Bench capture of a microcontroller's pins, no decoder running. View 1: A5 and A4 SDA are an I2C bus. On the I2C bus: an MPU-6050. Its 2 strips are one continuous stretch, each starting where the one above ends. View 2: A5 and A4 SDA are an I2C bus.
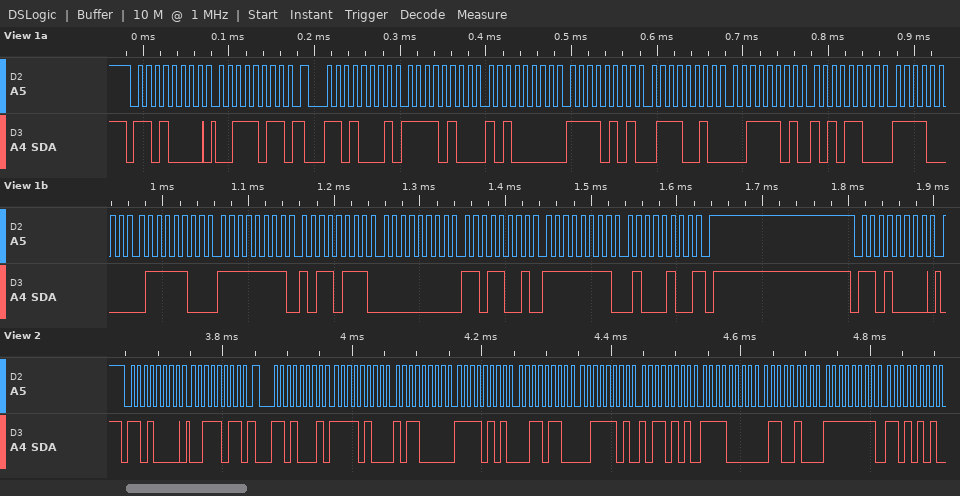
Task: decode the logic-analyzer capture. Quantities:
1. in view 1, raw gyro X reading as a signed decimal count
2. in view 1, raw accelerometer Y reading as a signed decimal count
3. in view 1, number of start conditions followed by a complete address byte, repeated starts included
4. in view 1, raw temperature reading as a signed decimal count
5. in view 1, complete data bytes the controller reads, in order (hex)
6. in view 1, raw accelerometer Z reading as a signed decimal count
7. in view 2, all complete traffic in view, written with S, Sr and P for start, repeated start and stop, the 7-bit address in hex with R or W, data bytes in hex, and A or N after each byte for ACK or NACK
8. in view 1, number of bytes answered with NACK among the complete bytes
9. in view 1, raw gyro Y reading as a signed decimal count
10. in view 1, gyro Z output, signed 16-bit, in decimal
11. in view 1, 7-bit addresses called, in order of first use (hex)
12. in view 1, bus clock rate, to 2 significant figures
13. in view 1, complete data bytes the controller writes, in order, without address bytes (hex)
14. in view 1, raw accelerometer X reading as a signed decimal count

-73
-2702
3
-3972
F4 A0 F5 72 3D AC F0 7C FF B7 00 D9 FF 44
15788
S 68W A 3B A Sr 68R A F4 A B0 A F5 A 36 A 3D A B5 A F0 A 64 A FF A D5 A
1
217
-188
0x68
100 kHz
3B
-2912
